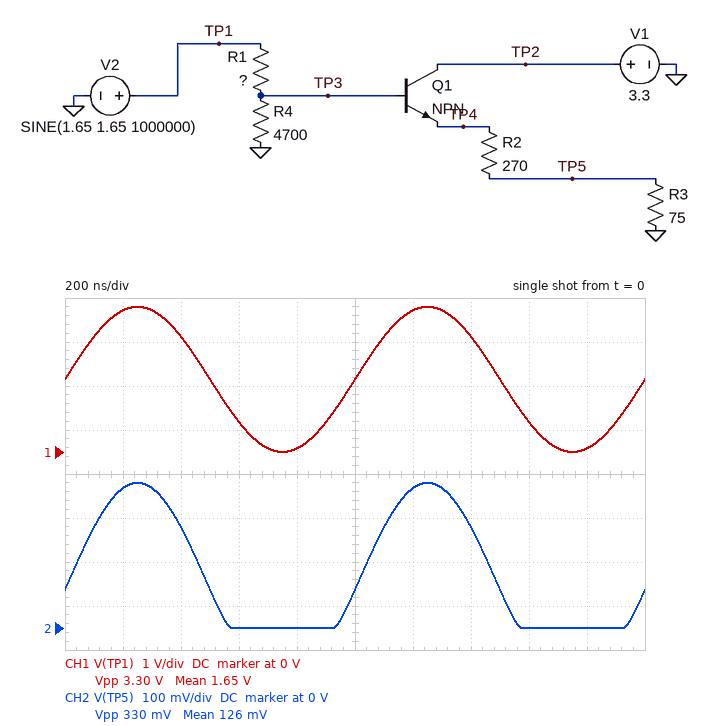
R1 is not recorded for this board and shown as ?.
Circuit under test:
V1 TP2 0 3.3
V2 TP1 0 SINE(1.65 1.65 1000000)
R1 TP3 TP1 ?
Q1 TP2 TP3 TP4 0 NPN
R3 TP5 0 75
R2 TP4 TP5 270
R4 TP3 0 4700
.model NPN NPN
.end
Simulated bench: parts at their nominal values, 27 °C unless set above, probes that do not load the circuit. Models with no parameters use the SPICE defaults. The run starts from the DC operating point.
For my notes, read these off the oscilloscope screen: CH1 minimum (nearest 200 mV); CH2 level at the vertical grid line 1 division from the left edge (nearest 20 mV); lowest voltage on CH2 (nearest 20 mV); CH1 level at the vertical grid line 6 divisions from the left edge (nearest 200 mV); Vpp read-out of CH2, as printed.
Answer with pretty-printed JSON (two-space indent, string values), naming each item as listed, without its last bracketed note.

{
  "CH1 minimum": "0 V",
  "CH2 level at the vertical grid line 1 division from the left edge": "320 mV",
  "lowest voltage on CH2": "0 V",
  "CH1 level at the vertical grid line 6 divisions from the left edge": "3.2 V",
  "Vpp read-out of CH2, as printed": "330 mV"
}
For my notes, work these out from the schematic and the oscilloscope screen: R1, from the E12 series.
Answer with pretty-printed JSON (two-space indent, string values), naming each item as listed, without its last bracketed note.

{
  "R1, from the E12 series": "1.8 kΩ"
}
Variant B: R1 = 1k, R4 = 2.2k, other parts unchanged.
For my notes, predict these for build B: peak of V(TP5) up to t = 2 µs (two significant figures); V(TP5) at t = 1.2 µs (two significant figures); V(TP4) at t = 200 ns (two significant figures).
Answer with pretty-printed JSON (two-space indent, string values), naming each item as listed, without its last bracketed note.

{
  "peak of V(TP5) up to t = 2 µs": "310 mV",
  "V(TP5) at t = 1.2 µs": "300 mV",
  "V(TP4) at t = 200 ns": "1.4 V"
}
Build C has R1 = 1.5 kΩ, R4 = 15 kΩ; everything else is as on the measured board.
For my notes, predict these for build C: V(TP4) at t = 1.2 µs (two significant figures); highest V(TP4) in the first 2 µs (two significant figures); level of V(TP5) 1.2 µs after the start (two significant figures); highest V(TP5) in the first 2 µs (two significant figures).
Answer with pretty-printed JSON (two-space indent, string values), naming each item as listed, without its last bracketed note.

{
  "V(TP4) at t = 1.2 µs": "2.0 V",
  "highest V(TP4) in the first 2 µs": "2.1 V",
  "level of V(TP5) 1.2 µs after the start": "440 mV",
  "highest V(TP5) in the first 2 µs": "460 mV"
}
